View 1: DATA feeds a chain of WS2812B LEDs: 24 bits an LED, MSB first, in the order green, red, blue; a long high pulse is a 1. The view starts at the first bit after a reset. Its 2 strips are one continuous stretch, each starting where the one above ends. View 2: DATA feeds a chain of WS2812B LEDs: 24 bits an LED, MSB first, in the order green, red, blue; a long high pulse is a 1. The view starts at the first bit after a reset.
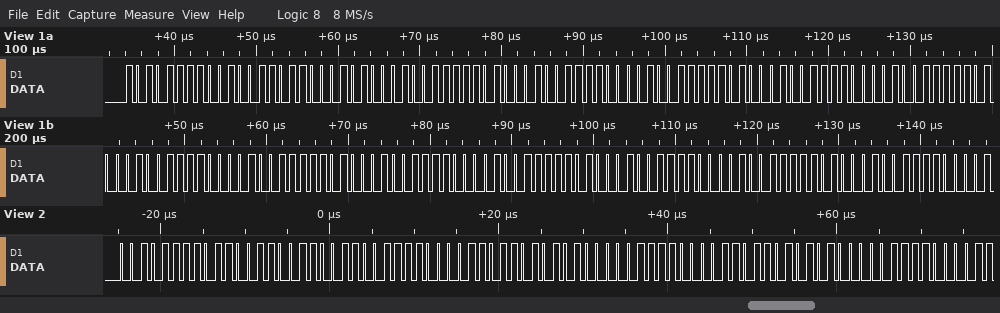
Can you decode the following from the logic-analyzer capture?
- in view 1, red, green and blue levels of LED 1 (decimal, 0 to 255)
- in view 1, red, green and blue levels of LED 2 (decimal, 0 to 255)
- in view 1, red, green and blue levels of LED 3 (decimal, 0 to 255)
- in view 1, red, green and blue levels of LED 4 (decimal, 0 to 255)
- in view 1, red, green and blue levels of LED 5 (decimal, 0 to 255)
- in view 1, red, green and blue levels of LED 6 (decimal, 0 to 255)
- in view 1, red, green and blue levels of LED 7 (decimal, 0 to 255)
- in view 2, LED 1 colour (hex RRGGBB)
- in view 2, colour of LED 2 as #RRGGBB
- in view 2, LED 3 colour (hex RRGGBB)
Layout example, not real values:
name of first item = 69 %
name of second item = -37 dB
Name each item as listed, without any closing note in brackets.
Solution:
in view 1, red, green and blue levels of LED 1 = 38, 175, 197
in view 1, red, green and blue levels of LED 2 = 232, 19, 158
in view 1, red, green and blue levels of LED 3 = 232, 19, 158
in view 1, red, green and blue levels of LED 4 = 232, 19, 158
in view 1, red, green and blue levels of LED 5 = 232, 19, 158
in view 1, red, green and blue levels of LED 6 = 232, 19, 158
in view 1, red, green and blue levels of LED 7 = 232, 19, 158
in view 2, LED 1 colour = #662F66
in view 2, colour of LED 2 as #RRGGBB = #6D7850
in view 2, LED 3 colour = #6D7850
